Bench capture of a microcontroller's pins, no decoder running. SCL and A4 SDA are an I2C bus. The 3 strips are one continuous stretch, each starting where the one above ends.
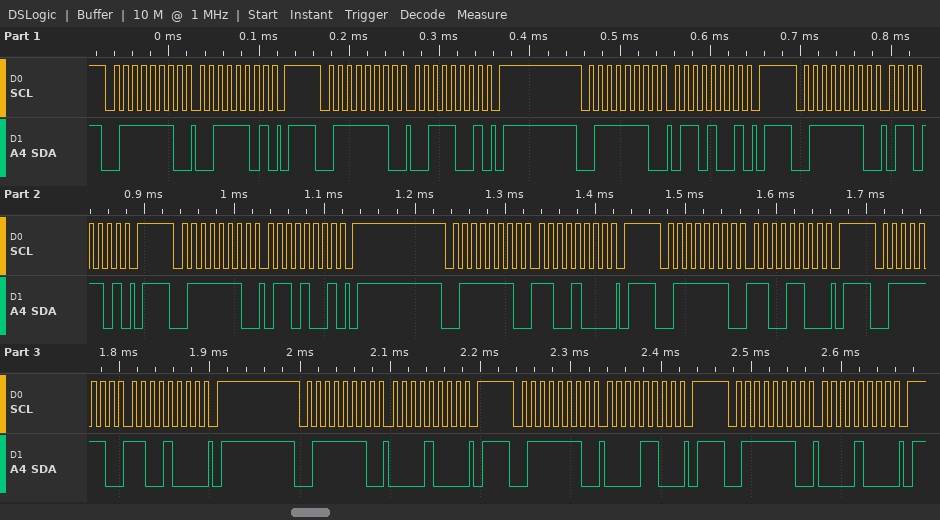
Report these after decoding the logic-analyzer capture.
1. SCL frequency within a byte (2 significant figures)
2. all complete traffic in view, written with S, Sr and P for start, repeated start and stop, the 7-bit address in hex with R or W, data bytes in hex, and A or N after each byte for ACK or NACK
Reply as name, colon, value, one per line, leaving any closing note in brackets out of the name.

SCL frequency within a byte: 100 kHz
all complete traffic in view, written with S, Sr and P for start, repeated start and stop, the 7-bit address in hex with R or W, data bytes in hex, and A or N after each byte for ACK or NACK: S 3FW A 3D A P S 3FW A 39 A P S 3FW A 69 A P S 3FW A 6D A P S 3FW A 69 A P S 3FW A C8 A P S 3FW A CC A P S 3FW A C8 A P S 3FW A 08 A P S 3FW A 0C A P S 3FW A 08 A P
